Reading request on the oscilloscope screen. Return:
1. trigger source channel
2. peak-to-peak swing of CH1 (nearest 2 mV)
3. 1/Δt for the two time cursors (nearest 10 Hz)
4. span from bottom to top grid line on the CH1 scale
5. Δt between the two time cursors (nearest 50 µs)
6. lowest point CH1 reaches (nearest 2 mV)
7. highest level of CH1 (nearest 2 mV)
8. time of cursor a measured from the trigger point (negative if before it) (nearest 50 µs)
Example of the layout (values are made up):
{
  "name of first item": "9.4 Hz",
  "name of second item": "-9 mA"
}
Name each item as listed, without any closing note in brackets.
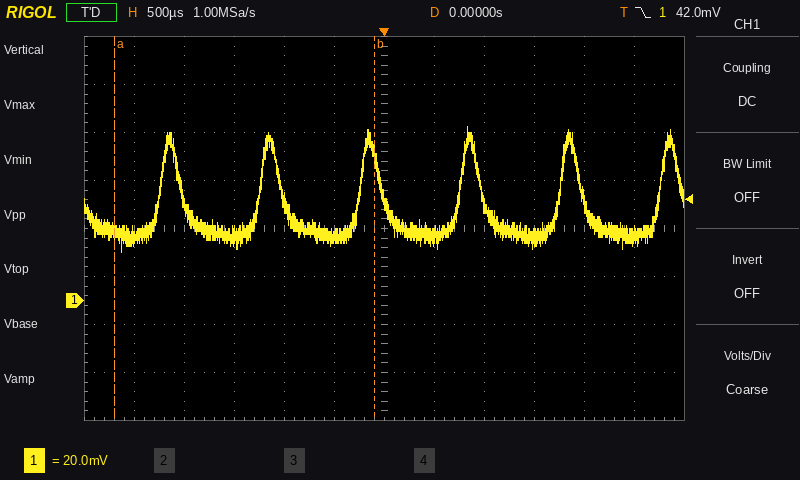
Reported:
{
  "trigger source channel": "CH1",
  "peak-to-peak swing of CH1": "52 mV",
  "1/Δt for the two time cursors": "380 Hz",
  "span from bottom to top grid line on the CH1 scale": "160 mV",
  "Δt between the two time cursors": "2.60 ms",
  "lowest point CH1 reaches": "20 mV",
  "highest level of CH1": "72 mV",
  "time of cursor a measured from the trigger point (negative if before it)": "-2.70 ms"
}
